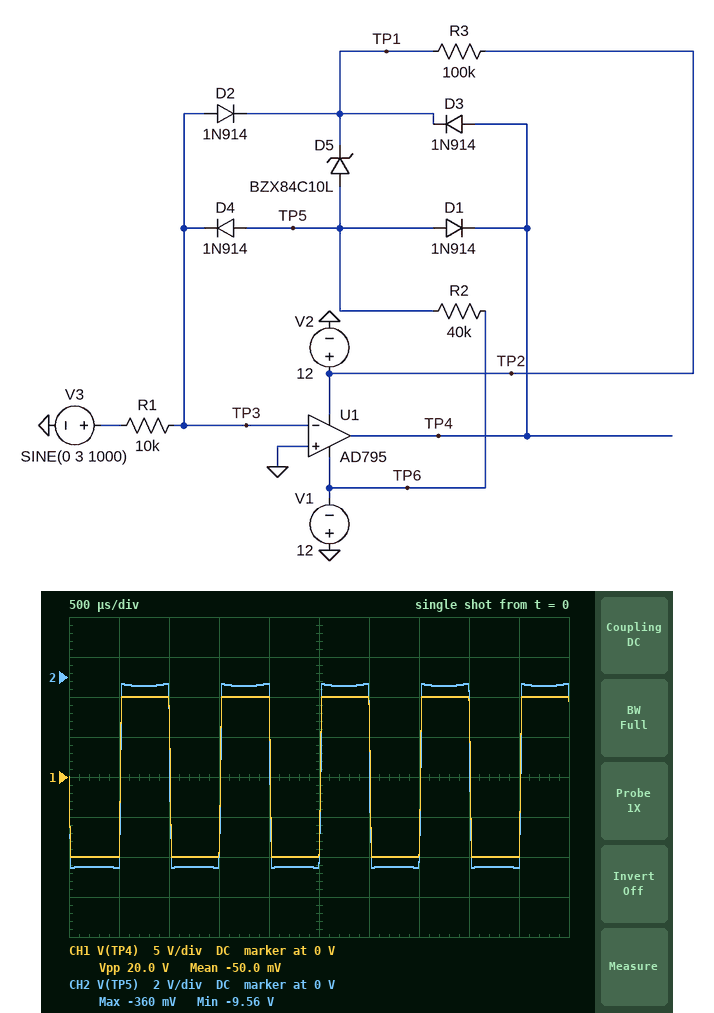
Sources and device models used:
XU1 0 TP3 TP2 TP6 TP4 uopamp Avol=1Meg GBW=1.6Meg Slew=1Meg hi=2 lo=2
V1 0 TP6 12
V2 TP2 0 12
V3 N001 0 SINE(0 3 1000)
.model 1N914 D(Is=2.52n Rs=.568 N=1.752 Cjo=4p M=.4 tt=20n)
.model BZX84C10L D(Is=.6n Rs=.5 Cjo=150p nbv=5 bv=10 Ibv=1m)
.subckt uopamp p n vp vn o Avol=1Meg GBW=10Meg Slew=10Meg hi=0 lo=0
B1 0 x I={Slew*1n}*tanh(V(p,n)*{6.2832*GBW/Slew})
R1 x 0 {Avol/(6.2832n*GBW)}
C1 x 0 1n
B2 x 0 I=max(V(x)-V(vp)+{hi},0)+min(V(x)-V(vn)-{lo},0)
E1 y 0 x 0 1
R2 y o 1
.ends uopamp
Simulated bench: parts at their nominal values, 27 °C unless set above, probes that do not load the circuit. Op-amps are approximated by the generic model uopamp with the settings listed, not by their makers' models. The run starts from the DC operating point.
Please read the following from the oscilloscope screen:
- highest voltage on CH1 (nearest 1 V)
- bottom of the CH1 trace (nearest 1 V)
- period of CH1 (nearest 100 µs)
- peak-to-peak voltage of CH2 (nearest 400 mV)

10 V
-10 V
1.0 ms
9.2 V
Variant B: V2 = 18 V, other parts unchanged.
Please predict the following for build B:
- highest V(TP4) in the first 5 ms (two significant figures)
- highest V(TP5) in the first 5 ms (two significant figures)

11 V
530 mV
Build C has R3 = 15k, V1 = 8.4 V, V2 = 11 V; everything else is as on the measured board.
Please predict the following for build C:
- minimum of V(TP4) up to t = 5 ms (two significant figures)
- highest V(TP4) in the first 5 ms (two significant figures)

-6.4 V
9.0 V
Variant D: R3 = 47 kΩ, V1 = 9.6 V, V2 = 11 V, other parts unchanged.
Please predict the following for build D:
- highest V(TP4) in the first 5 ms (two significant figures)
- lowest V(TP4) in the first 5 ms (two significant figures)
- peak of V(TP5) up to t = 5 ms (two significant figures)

9.0 V
-7.6 V
-1.3 V
